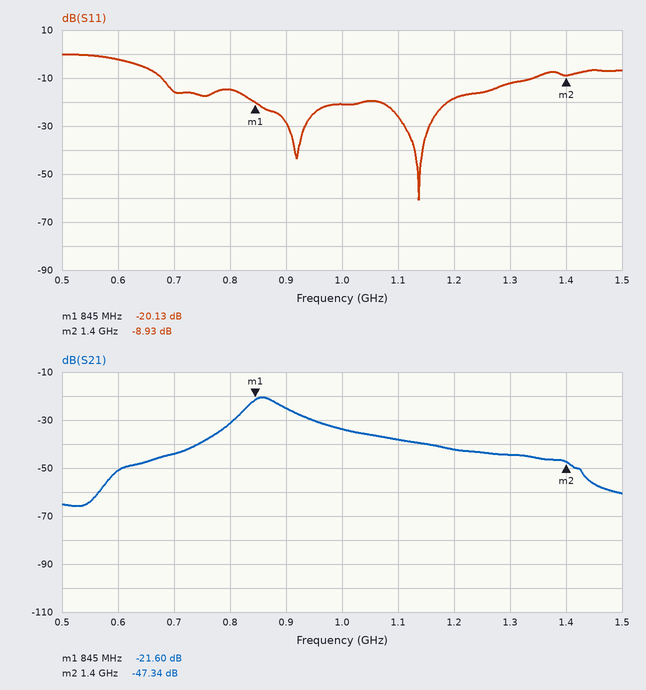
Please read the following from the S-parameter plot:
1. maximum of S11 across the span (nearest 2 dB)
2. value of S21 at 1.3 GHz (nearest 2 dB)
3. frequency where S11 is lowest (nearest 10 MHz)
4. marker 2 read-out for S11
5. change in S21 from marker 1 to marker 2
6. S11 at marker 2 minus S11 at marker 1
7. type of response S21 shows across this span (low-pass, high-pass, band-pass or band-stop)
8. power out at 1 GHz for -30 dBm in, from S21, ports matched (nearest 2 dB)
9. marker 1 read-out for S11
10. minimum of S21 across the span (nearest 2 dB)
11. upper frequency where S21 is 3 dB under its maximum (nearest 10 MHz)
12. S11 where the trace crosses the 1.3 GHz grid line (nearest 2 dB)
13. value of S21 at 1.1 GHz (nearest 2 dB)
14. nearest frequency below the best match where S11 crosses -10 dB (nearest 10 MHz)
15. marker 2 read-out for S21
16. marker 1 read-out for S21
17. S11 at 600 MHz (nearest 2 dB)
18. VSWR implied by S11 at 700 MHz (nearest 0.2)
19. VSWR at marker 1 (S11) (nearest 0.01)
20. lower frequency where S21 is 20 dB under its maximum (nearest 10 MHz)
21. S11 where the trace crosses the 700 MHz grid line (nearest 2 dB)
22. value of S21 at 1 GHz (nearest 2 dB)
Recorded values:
0 dB
-44 dB
1.14 GHz
-8.93 dB
-25.74 dB
11.20 dB
band-pass
-64 dBm
-20.13 dB
-66 dB
890 MHz
-12 dB
-38 dB
680 MHz
-47.34 dB
-21.60 dB
-2 dB
1.4
1.22
740 MHz
-16 dB
-34 dB
